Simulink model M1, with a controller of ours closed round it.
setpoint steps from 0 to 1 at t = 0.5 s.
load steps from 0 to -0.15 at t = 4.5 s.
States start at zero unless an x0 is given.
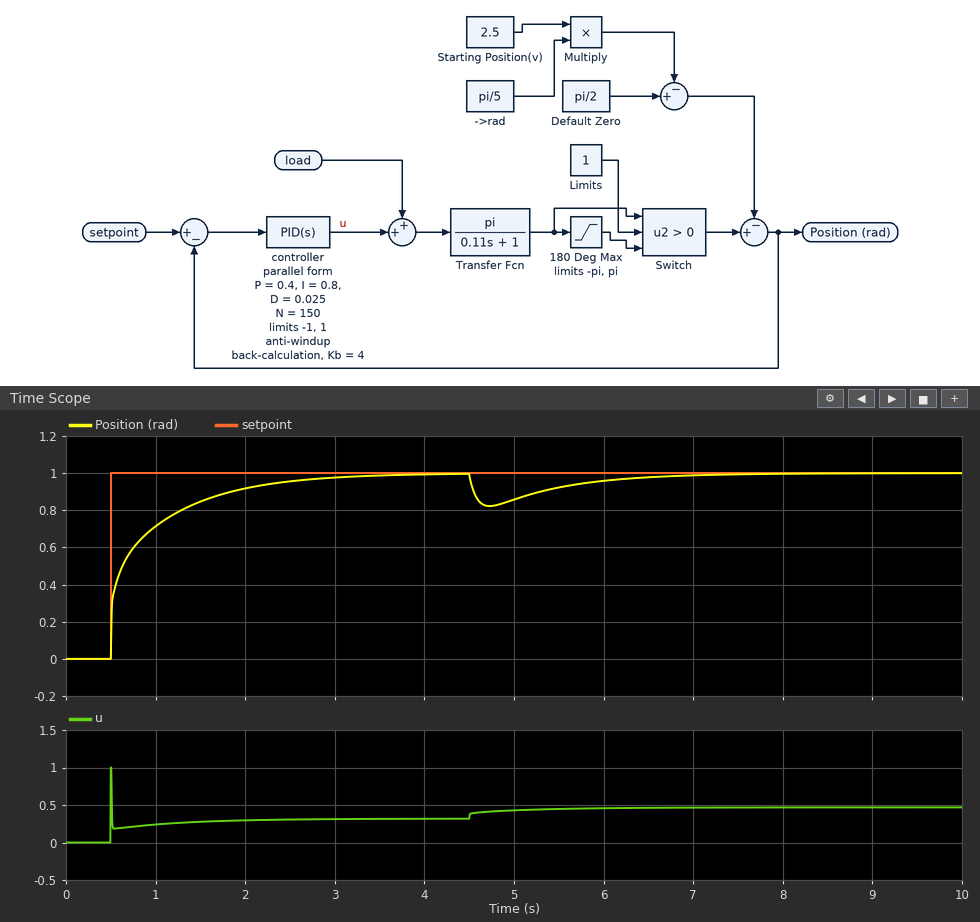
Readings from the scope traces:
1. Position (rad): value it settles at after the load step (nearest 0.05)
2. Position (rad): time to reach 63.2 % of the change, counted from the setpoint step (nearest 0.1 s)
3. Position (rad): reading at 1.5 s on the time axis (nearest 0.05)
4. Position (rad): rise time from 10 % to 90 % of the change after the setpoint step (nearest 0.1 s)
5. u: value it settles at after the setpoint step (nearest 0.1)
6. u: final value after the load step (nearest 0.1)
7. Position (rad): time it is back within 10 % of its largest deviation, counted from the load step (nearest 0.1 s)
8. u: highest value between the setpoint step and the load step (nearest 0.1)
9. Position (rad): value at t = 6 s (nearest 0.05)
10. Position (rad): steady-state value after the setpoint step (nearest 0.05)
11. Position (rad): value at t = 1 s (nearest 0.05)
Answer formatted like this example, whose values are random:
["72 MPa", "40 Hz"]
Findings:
["1.00", "0.3 s", "0.85", "1.3 s", "0.3", "0.5", "2.2 s", "1.0", "0.95", "1.00", "0.70"]
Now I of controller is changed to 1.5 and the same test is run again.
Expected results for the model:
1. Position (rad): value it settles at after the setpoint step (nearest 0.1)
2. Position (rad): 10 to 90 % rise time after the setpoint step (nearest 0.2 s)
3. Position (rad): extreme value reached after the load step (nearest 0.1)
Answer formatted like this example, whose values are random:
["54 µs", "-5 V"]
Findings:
["1.0", "0.6 s", "0.8"]
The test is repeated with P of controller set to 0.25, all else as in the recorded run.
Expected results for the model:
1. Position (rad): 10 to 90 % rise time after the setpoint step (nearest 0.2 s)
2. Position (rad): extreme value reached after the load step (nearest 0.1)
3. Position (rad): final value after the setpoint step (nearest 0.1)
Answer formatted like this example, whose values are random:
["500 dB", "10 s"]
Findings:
["1.2 s", "0.8", "1.0"]
